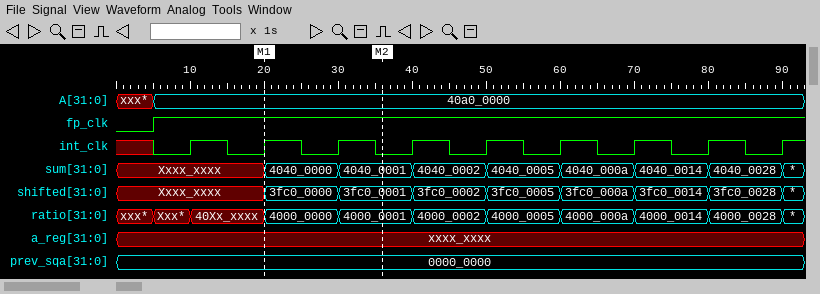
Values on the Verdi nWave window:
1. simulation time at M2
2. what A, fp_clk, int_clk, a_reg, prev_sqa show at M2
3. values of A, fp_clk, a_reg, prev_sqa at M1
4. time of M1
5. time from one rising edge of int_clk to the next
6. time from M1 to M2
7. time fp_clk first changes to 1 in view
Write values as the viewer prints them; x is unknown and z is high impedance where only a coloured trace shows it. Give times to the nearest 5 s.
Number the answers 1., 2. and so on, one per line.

1. 35 s
2. A=40a0_0000, fp_clk=1, int_clk=0, a_reg=xxxx_xxxx, prev_sqa=0000_0000
3. A=40a0_0000, fp_clk=1, a_reg=xxxx_xxxx, prev_sqa=0000_0000
4. 20 s
5. 10 s
6. 15 s
7. 5 s
